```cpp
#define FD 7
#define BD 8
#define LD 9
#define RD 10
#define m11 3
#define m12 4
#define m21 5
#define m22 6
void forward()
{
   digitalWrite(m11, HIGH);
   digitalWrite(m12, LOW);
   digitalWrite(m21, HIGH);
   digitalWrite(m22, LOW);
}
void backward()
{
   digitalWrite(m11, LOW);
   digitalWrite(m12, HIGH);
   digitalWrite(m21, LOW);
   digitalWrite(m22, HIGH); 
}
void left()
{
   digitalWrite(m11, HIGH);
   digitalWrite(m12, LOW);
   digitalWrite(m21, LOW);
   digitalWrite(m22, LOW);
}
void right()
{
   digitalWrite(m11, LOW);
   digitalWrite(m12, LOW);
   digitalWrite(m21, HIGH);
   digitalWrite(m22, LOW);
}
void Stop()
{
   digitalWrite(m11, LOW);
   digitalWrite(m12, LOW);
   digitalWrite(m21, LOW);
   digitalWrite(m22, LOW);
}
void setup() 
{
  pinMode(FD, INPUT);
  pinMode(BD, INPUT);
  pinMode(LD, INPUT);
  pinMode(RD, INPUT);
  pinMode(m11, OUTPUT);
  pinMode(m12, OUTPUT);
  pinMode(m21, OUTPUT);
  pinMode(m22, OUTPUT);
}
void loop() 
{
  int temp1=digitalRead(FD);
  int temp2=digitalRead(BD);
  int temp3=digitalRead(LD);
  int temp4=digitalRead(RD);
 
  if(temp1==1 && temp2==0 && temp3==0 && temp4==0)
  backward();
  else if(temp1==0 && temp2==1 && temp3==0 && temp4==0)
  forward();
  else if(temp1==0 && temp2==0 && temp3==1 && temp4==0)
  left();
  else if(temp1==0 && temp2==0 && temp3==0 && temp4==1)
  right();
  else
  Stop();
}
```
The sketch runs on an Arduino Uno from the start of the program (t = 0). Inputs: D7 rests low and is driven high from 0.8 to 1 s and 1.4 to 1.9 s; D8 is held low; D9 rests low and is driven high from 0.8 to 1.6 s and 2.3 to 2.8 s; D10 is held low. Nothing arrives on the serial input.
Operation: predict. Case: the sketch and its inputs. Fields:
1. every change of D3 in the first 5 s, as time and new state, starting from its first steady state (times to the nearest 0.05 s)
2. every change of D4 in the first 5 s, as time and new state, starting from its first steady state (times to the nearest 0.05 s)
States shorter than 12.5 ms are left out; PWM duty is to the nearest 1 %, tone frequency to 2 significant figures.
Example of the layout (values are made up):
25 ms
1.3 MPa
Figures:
0 s low; 1 s high; 1.4 s low; 2.3 s high; 2.8 s low
0 s low; 1.6 s high; 1.9 s low
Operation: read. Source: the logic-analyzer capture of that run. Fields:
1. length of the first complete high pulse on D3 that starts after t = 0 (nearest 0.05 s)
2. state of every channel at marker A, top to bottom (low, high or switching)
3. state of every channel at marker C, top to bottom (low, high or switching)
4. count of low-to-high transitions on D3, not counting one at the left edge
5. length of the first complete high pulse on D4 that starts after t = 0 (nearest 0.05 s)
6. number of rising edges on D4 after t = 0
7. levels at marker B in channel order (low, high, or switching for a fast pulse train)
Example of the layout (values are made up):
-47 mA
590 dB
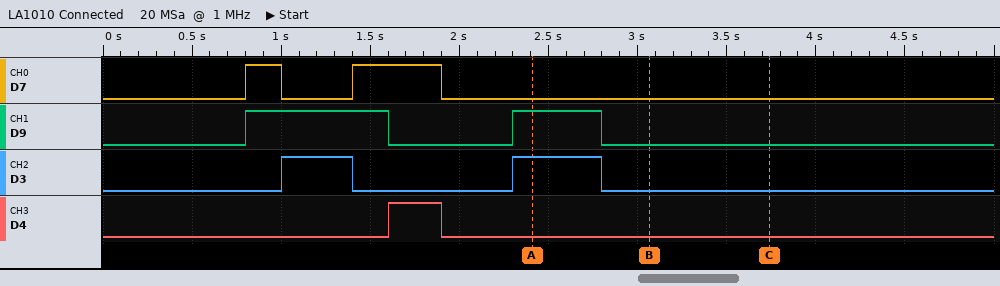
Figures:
0.40 s
D7 low, D9 high, D3 high, D4 low
D7 low, D9 low, D3 low, D4 low
2
0.30 s
1
D7 low, D9 low, D3 low, D4 low
